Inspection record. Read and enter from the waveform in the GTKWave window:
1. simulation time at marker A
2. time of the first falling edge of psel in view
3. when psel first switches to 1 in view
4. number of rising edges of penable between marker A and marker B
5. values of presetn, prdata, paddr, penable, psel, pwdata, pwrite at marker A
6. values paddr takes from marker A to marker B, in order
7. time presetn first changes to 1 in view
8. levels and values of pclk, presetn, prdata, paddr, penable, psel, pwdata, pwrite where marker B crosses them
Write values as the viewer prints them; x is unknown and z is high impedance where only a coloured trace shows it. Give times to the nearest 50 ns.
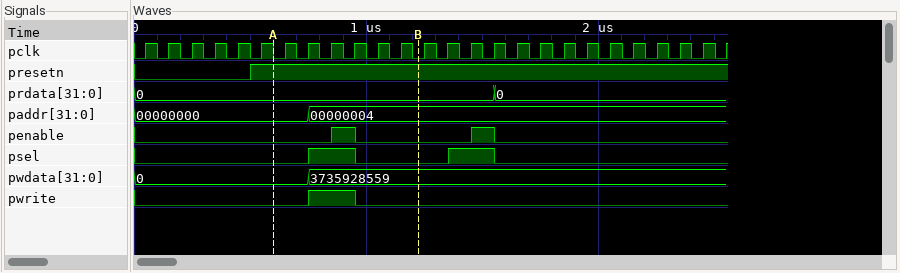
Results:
600 ns
950 ns
750 ns
1
presetn=1, prdata=0, paddr=00000000, penable=0, psel=0, pwdata=0, pwrite=0
00000000, 00000004
500 ns
pclk=0, presetn=1, prdata=0, paddr=00000004, penable=0, psel=0, pwdata=3735928559, pwrite=0
